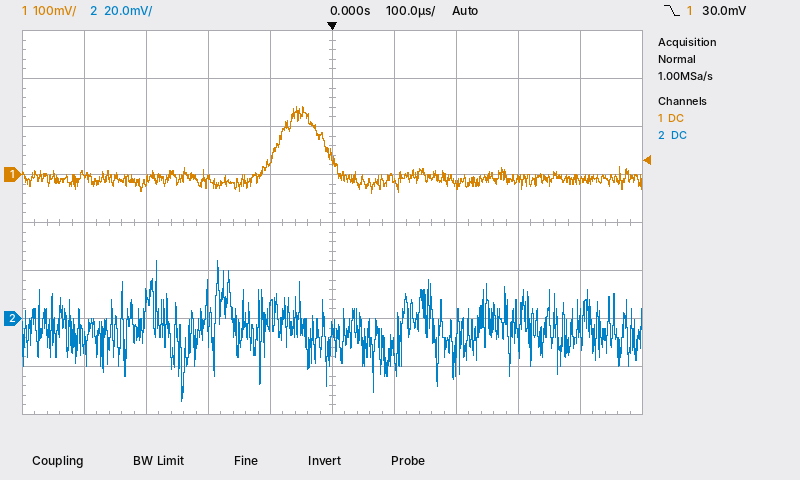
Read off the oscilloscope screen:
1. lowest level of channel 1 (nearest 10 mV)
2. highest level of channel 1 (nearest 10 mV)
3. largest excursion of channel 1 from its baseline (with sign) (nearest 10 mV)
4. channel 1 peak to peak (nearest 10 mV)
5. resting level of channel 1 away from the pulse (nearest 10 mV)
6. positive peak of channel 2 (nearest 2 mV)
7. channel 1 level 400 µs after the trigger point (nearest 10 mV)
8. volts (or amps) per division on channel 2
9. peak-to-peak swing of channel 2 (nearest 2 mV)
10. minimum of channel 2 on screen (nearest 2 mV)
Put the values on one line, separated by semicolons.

-40 mV; 140 mV; +150 mV; 180 mV; -10 mV; 24 mV; -10 mV; 20 mV; 58 mV; -34 mV
